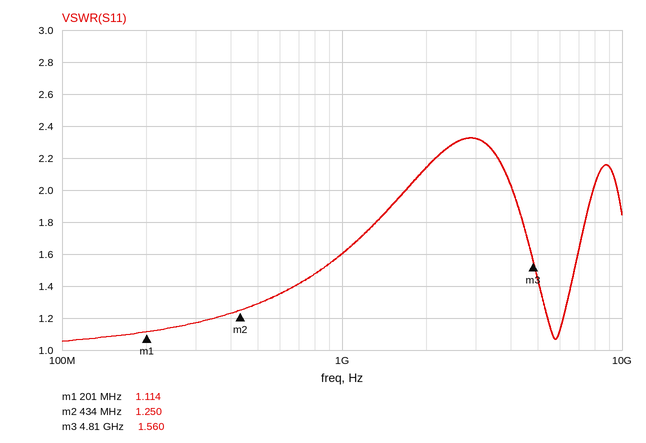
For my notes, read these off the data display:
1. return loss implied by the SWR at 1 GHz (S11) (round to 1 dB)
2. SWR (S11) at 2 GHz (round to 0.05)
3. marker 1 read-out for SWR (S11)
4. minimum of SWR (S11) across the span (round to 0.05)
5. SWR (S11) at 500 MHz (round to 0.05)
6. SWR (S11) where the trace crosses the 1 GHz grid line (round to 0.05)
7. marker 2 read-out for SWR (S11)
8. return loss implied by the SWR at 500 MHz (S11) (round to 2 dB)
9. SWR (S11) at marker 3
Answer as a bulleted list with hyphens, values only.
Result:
- 13 dB
- 2.15
- 1.114
- 1.05
- 1.30
- 1.60
- 1.250
- 18 dB
- 1.560
